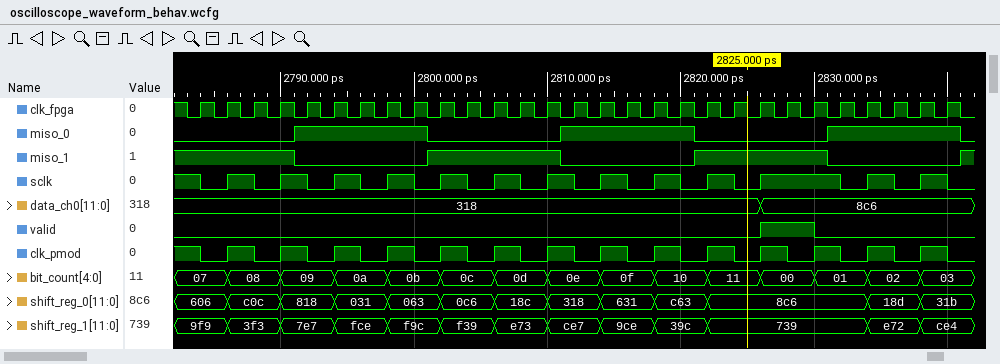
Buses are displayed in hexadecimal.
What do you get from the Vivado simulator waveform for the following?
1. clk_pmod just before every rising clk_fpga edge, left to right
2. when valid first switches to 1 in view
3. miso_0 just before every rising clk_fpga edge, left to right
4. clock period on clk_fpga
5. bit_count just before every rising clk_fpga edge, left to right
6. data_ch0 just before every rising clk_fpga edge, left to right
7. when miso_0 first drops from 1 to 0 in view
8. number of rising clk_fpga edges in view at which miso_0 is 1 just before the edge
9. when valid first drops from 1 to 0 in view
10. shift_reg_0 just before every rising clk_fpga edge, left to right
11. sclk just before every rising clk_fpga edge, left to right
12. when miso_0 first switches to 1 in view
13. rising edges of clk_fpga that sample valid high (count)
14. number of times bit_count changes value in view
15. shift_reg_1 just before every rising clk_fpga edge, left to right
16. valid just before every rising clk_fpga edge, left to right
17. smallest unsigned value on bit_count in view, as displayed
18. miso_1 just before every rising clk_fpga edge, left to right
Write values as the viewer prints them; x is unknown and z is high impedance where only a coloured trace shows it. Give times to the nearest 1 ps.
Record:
1 0 1 0 1 0 1 0 1 0 1 0 1 0 1 0 1 0 1 0 1 0 1 0 1 0 1 0 1
2826 ps
0 0 0 0 1 1 1 1 1 0 0 0 0 0 1 1 1 1 1 0 0 0 0 0 1 1 1 1 1
2 ps
07, 07, 08, 08, 09, 09, 0a, 0a, 0b, 0b, 0c, 0c, 0d, 0d, 0e, 0e, 0f, 0f, 10, 10, 11, 11, 00, 00, 01, 01, 02, 02, 03
318, 318, 318, 318, 318, 318, 318, 318, 318, 318, 318, 318, 318, 318, 318, 318, 318, 318, 318, 318, 318, 318, 8c6, 8c6, 8c6, 8c6, 8c6, 8c6, 8c6
2801 ps
15
2830 ps
606, 606, c0c, c0c, 818, 818, 031, 031, 063, 063, 0c6, 0c6, 18c, 18c, 318, 318, 631, 631, c63, c63, 8c6, 8c6, 8c6, 8c6, 8c6, 8c6, 18d, 18d, 31b
1 0 1 0 1 0 1 0 1 0 1 0 1 0 1 0 1 0 1 0 1 0 1 1 1 0 1 0 1
2791 ps
2
14
9f9, 9f9, 3f3, 3f3, 7e7, 7e7, fce, fce, f9c, f9c, f39, f39, e73, e73, ce7, ce7, 9ce, 9ce, 39c, 39c, 739, 739, 739, 739, 739, 739, e72, e72, ce4
0 0 0 0 0 0 0 0 0 0 0 0 0 0 0 0 0 0 0 0 0 0 1 1 0 0 0 0 0
00
1 1 1 1 0 0 0 0 0 1 1 1 1 1 0 0 0 0 0 1 1 1 1 1 0 0 0 0 0
